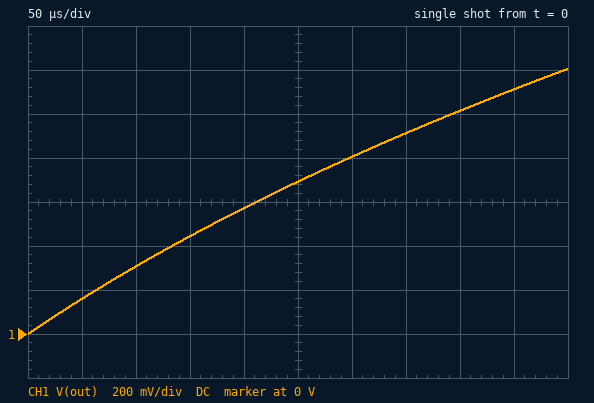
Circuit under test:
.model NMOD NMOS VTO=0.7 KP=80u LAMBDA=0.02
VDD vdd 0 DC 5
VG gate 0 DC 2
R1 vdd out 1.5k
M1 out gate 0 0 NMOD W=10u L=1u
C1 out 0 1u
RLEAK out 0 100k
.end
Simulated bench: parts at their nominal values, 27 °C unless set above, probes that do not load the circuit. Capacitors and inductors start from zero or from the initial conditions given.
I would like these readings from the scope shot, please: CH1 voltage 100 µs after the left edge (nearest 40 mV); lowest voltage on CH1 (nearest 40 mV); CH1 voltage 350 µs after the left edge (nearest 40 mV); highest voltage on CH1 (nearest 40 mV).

320 mV
0 V
920 mV
1.20 V
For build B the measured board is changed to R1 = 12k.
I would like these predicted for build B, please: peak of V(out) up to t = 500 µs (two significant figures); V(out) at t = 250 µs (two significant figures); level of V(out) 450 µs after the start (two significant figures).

160 mV
91 mV
150 mV
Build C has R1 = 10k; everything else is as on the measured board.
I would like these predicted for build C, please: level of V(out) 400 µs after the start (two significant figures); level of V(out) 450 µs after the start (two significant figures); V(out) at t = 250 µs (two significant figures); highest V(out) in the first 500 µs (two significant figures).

160 mV
180 mV
110 mV
190 mV
